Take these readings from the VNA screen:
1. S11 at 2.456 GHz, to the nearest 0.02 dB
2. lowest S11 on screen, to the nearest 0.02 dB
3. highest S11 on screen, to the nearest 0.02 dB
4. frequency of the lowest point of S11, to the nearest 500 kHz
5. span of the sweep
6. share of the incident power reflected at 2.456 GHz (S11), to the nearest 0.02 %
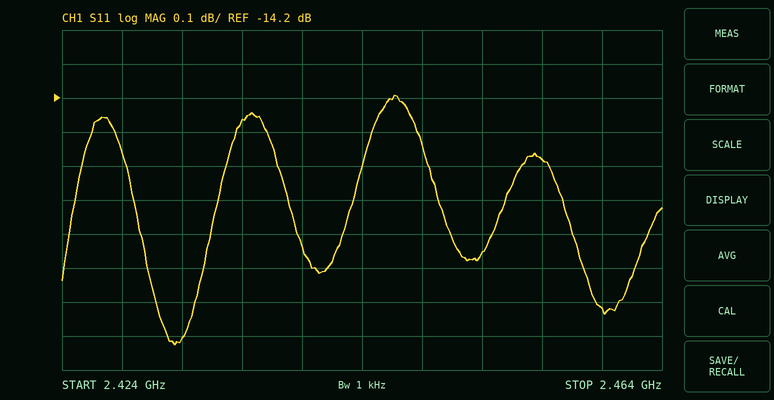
-14.38 dB
-14.92 dB
-14.20 dB
2.4315 GHz
40 MHz
3.64 %
